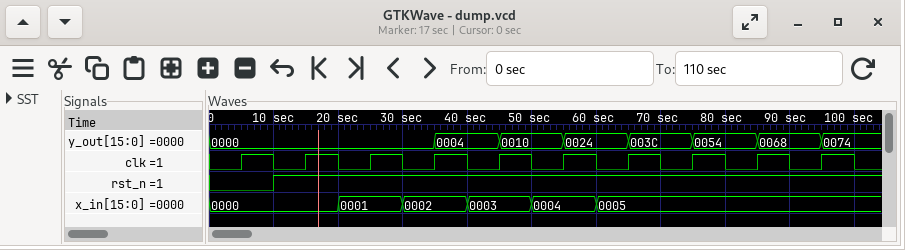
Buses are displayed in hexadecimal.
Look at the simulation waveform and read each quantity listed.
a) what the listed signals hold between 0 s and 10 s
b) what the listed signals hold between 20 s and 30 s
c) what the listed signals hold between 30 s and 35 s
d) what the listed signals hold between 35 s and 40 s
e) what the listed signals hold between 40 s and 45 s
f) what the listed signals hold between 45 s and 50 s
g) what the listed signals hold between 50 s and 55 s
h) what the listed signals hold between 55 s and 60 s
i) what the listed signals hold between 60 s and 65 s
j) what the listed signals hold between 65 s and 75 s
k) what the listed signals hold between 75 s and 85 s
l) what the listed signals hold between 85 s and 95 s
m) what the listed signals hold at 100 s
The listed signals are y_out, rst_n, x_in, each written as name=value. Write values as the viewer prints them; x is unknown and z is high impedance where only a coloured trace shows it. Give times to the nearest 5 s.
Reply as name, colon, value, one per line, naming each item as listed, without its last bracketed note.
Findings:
what the listed signals hold between 0 s and 10 s: y_out=0000, rst_n=0, x_in=0000
what the listed signals hold between 20 s and 30 s: y_out=0000, rst_n=1, x_in=0001
what the listed signals hold between 30 s and 35 s: y_out=0000, rst_n=1, x_in=0002
what the listed signals hold between 35 s and 40 s: y_out=0004, rst_n=1, x_in=0002
what the listed signals hold between 40 s and 45 s: y_out=0004, rst_n=1, x_in=0003
what the listed signals hold between 45 s and 50 s: y_out=0010, rst_n=1, x_in=0003
what the listed signals hold between 50 s and 55 s: y_out=0010, rst_n=1, x_in=0004
what the listed signals hold between 55 s and 60 s: y_out=0024, rst_n=1, x_in=0004
what the listed signals hold between 60 s and 65 s: y_out=0024, rst_n=1, x_in=0005
what the listed signals hold between 65 s and 75 s: y_out=003C, rst_n=1, x_in=0005
what the listed signals hold between 75 s and 85 s: y_out=0054, rst_n=1, x_in=0005
what the listed signals hold between 85 s and 95 s: y_out=0068, rst_n=1, x_in=0005
what the listed signals hold at 100 s: y_out=0074, rst_n=1, x_in=0005
